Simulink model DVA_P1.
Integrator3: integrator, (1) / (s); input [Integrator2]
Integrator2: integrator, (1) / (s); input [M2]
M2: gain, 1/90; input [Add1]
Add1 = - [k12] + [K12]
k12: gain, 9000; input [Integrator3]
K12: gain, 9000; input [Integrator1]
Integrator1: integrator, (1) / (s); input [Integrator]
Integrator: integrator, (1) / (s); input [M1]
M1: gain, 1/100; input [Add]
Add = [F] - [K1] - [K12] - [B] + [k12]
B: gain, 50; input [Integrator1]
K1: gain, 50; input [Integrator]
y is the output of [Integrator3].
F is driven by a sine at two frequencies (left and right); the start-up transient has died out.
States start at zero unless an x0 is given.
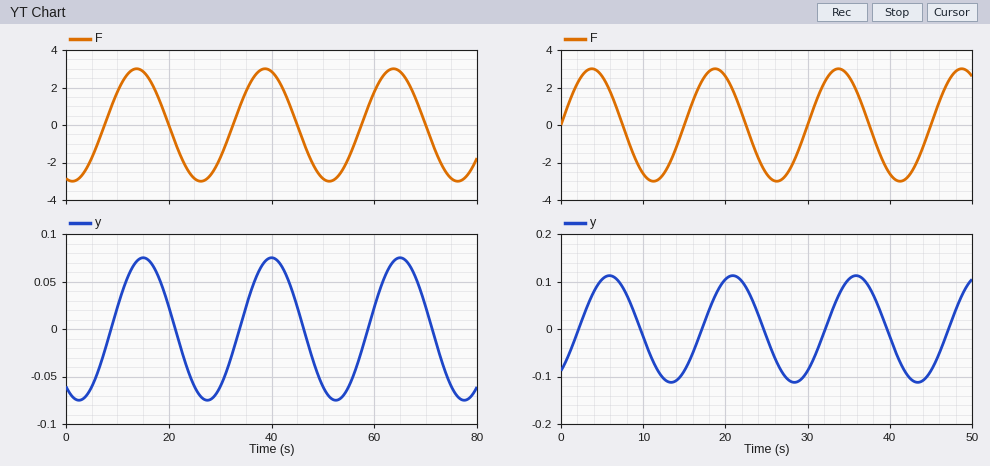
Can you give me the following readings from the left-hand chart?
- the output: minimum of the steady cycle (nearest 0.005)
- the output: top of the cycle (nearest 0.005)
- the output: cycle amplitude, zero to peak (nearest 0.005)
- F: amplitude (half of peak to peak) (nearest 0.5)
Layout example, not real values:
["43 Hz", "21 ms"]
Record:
["-0.075", "0.075", "0.075", "3.0"]
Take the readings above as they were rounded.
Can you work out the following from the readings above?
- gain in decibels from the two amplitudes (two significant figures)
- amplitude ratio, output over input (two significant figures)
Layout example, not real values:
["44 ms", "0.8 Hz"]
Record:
["-32 dB", "0.025"]
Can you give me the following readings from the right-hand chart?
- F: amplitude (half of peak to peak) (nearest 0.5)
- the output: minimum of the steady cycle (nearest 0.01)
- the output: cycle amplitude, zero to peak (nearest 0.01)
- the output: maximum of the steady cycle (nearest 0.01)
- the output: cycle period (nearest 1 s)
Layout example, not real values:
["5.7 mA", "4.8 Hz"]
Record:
["3.0", "-0.11", "0.11", "0.11", "15 s"]
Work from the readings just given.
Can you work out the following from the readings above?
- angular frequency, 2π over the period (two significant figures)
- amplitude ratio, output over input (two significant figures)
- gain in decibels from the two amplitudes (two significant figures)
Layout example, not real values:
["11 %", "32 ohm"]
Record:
["0.42 rad/s", "0.037", "-29 dB"]
